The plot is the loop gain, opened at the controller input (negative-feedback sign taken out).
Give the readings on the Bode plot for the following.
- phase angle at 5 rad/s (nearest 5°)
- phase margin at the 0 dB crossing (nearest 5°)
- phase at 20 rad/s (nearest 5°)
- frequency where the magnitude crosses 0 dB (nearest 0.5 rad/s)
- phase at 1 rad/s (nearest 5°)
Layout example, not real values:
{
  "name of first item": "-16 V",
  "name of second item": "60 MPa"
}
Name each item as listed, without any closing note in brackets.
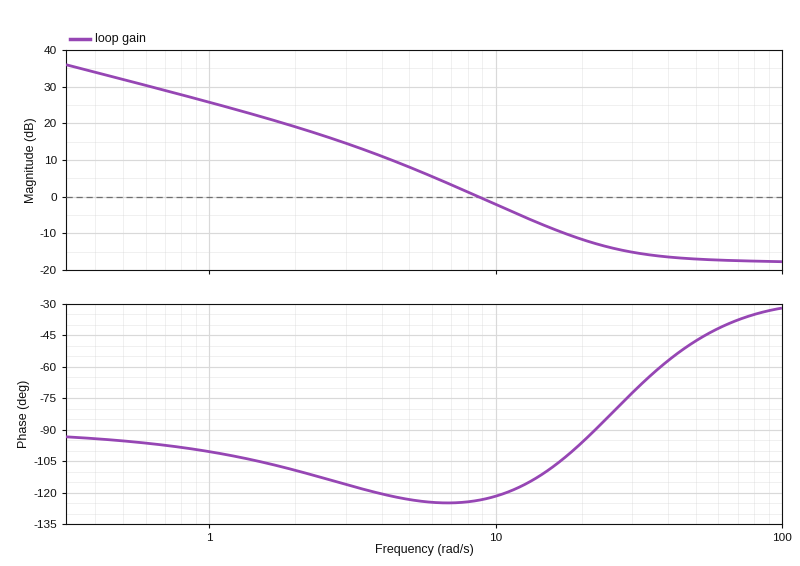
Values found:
{
  "phase angle at 5 rad/s": "-125°",
  "phase margin at the 0 dB crossing": "55°",
  "phase at 20 rad/s": "-95°",
  "frequency where the magnitude crosses 0 dB": "8.5 rad/s",
  "phase at 1 rad/s": "-100°"
}
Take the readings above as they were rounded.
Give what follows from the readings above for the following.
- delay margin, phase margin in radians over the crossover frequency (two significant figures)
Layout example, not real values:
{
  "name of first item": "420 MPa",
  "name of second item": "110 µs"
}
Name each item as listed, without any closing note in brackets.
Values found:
{
  "delay margin, phase margin in radians over the crossover frequency": "0.11 s"
}
